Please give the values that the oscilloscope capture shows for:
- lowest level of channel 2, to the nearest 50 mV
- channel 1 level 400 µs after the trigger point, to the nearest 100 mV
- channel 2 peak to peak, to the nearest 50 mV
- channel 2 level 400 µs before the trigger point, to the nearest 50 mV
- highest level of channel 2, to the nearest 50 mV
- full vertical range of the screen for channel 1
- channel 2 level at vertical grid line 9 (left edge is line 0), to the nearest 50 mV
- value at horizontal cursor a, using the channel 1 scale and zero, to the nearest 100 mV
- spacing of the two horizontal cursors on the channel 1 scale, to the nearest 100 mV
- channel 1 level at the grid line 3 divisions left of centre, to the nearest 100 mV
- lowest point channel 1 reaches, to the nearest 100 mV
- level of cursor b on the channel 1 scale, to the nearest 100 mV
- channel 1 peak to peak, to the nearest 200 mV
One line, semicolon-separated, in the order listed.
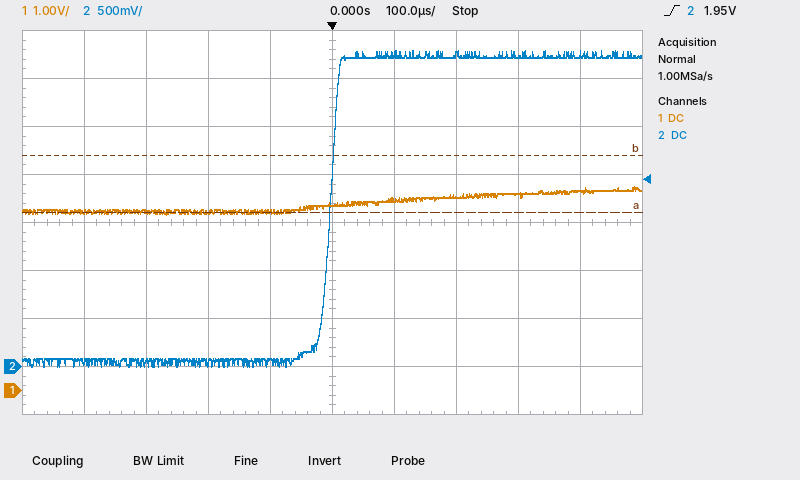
0 mV; 4.2 V; 3.30 V; 50 mV; 3.30 V; 8 V; 3.25 V; 3.7 V; 1.2 V; 3.7 V; 3.7 V; 4.9 V; 600 mV
